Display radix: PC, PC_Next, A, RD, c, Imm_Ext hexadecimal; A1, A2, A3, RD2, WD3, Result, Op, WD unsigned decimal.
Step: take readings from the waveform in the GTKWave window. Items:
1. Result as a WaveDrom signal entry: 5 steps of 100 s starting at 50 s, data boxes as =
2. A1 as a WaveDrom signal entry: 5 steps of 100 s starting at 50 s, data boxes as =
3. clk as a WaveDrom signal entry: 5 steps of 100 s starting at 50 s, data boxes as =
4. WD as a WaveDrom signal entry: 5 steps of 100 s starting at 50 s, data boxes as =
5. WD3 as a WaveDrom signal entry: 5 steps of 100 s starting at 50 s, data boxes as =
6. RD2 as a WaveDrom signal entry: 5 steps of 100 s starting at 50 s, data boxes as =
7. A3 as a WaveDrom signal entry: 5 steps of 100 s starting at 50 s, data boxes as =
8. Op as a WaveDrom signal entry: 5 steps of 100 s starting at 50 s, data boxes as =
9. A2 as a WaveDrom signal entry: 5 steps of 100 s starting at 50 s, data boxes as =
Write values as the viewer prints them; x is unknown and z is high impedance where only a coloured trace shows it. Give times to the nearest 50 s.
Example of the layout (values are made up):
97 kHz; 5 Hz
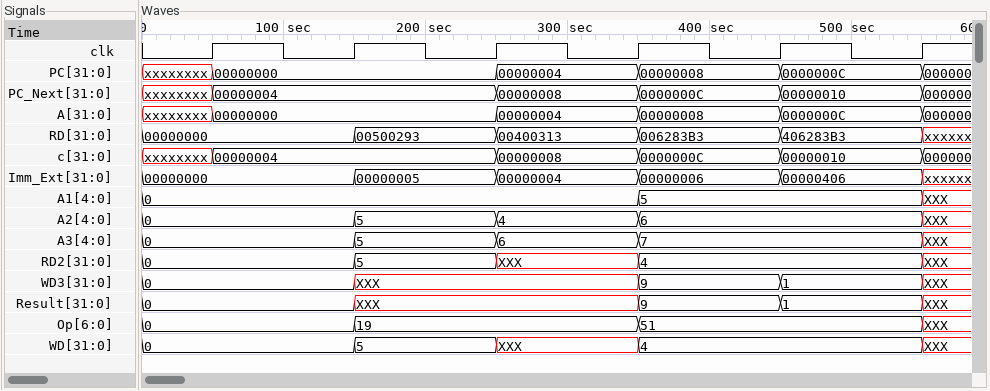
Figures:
{name: 'Result', wave: '=x.==', data: '0 9 1'}; {name: 'A1', wave: '=..=.', data: '0 5'}; {name: 'clk', wave: 'p....'}; {name: 'WD', wave: '==x=.', data: '0 5 4'}; {name: 'WD3', wave: '=x.==', data: '0 9 1'}; {name: 'RD2', wave: '==x=.', data: '0 5 4'}; {name: 'A3', wave: '====.', data: '0 5 6 7'}; {name: 'Op', wave: '==.=.', data: '0 19 51'}; {name: 'A2', wave: '====.', data: '0 5 4 6'}
